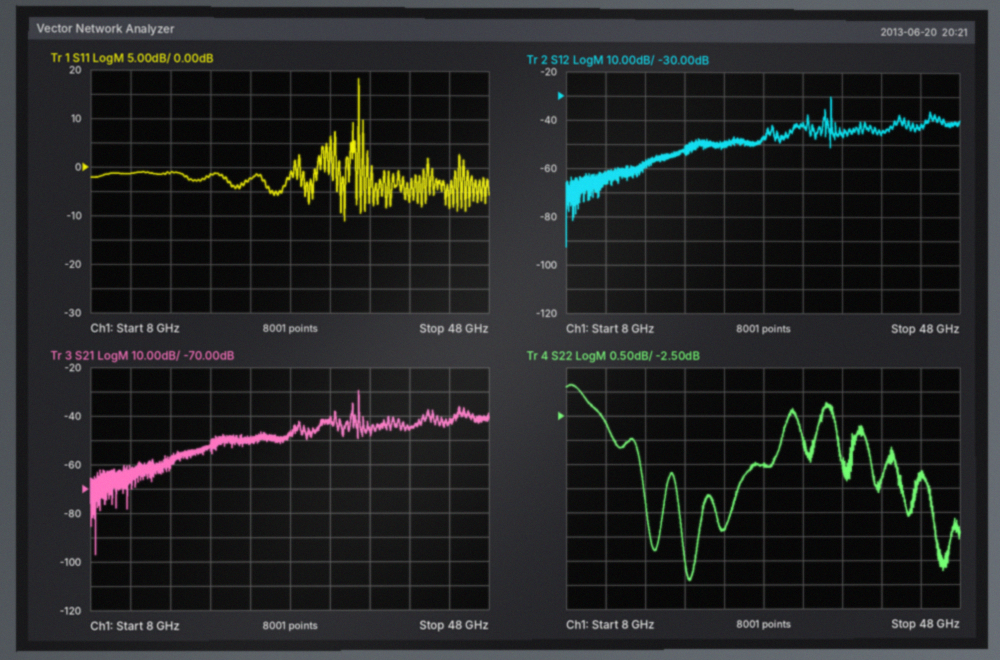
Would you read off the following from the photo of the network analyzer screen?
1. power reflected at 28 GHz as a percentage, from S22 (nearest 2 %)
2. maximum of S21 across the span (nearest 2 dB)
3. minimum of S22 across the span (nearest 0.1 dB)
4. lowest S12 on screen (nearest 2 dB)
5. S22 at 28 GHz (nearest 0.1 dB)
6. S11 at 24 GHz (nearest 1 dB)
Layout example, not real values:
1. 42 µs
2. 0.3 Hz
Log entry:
1. 44 %
2. -30 dB
3. -5.9 dB
4. -92 dB
5. -3.5 dB
6. -2 dB
